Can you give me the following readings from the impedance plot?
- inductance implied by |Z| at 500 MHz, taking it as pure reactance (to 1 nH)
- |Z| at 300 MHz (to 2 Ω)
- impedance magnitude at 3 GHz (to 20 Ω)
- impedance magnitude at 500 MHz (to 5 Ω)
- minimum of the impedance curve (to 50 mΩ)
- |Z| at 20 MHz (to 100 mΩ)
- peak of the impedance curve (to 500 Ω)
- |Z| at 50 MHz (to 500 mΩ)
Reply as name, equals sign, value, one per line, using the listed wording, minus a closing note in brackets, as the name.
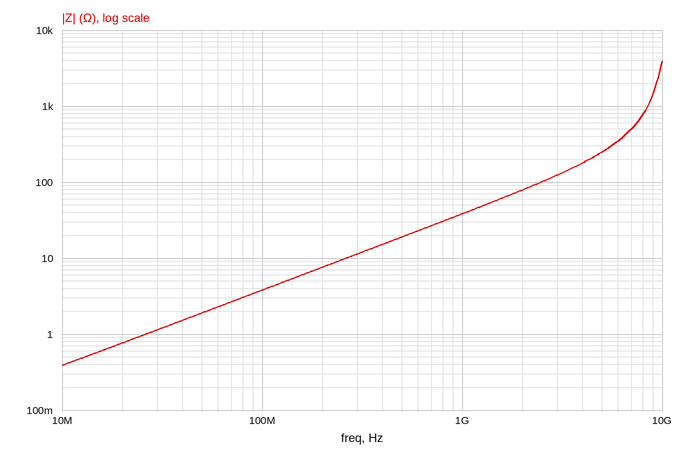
inductance implied by |Z| at 500 MHz, taking it as pure reactance = 6 nH
|Z| at 300 MHz = 12 Ω
impedance magnitude at 3 GHz = 120 Ω
impedance magnitude at 500 MHz = 20 Ω
minimum of the impedance curve = 400 mΩ
|Z| at 20 MHz = 800 mΩ
peak of the impedance curve = 4.0 kΩ
|Z| at 50 MHz = 2.0 Ω
